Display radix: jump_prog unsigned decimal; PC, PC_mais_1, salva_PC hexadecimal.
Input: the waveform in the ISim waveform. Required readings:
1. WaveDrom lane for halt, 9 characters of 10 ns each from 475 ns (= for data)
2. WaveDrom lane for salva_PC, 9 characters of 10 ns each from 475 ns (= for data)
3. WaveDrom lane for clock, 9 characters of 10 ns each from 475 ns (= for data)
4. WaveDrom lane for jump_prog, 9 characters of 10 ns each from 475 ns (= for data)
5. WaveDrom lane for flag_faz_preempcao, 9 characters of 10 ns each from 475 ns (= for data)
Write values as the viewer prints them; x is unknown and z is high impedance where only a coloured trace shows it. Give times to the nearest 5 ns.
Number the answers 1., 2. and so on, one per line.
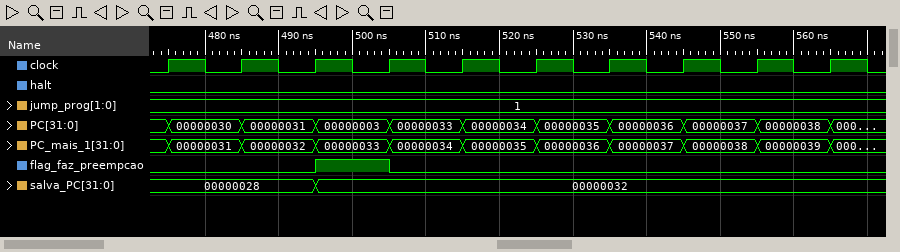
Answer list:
1. {name: 'halt', wave: '0........'}
2. {name: 'salva_PC', wave: '=.=......', data: '00000028 00000032'}
3. {name: 'clock', wave: 'p........'}
4. {name: 'jump_prog', wave: '=........', data: '1'}
5. {name: 'flag_faz_preempcao', wave: '0.10.....'}
